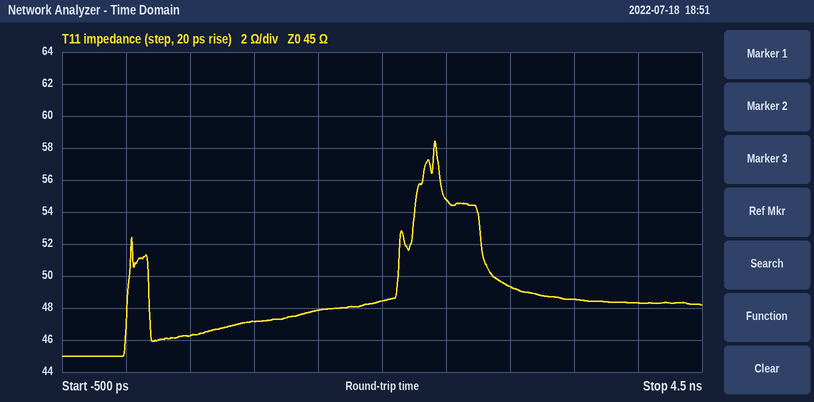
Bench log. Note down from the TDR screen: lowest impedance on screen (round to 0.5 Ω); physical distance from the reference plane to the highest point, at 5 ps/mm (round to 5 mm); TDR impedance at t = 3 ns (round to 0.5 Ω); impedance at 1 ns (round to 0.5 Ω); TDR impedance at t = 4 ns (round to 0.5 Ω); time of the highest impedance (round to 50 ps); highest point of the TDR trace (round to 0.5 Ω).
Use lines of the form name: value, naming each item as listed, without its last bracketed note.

lowest impedance on screen: 45.0 Ω
physical distance from the reference plane to the highest point, at 5 ps/mm: 240 mm
TDR impedance at t = 3 ns: 49.5 Ω
impedance at 1 ns: 47.0 Ω
TDR impedance at t = 4 ns: 48.5 Ω
time of the highest impedance: 2.40 ns
highest point of the TDR trace: 58.5 Ω
